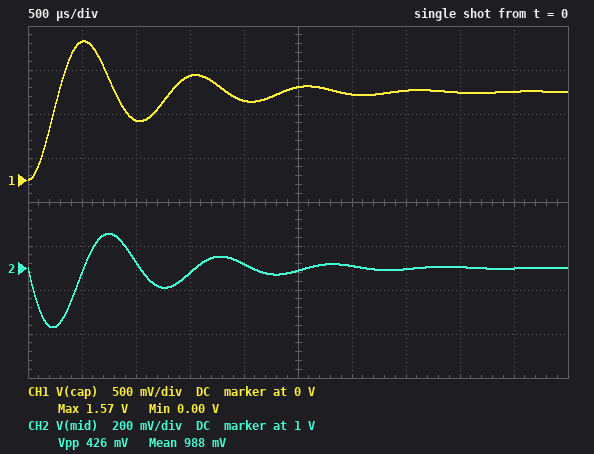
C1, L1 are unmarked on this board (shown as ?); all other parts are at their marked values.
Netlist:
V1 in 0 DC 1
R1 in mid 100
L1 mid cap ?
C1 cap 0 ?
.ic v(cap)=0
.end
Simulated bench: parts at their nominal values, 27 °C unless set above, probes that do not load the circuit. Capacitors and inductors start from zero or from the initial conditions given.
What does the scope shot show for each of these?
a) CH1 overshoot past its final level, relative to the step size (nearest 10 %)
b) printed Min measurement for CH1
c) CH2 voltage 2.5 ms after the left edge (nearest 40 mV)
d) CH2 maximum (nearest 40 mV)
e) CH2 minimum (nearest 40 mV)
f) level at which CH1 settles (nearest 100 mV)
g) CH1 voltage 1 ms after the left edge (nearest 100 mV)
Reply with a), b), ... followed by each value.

a) 60 %
b) 0.00 V
c) 1.00 V
d) 1.16 V
e) 720 mV
f) 1.0 V
g) 700 mV
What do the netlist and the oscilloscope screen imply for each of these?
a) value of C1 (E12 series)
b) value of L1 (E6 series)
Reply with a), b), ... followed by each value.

a) 560 nF
b) 47 mH
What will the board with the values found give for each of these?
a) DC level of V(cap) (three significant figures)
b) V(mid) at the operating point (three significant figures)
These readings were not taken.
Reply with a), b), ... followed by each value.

a) 1.00 V
b) 1.00 V
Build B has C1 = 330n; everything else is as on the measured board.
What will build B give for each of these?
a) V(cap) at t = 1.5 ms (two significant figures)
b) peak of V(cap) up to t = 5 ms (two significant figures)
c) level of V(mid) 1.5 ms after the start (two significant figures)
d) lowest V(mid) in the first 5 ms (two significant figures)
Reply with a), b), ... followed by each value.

a) 850 mV
b) 1.7 V
c) 1.0 V
d) 780 mV
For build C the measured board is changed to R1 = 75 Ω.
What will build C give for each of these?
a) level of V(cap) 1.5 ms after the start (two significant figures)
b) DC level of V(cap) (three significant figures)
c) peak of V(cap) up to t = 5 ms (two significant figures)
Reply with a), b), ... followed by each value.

a) 1.3 V
b) 1.00 V
c) 1.7 V
